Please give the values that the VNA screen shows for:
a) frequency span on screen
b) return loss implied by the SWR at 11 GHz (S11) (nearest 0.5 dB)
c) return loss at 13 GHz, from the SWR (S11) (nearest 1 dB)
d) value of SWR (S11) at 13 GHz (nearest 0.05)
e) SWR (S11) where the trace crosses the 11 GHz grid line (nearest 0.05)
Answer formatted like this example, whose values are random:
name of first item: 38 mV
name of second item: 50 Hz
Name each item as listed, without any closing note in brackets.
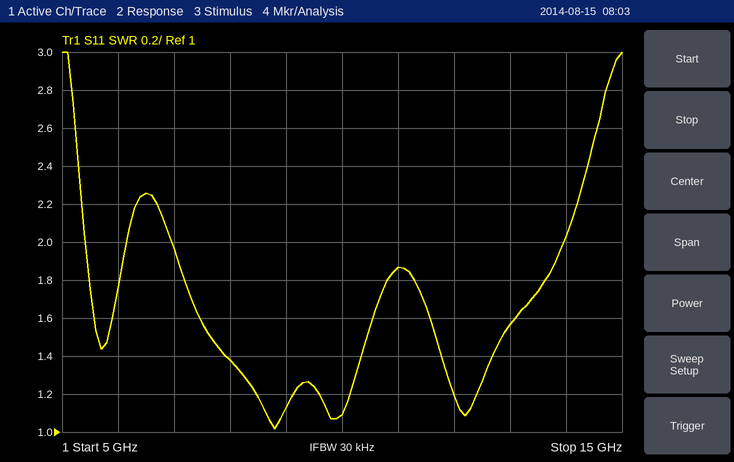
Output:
frequency span on screen: 10 GHz
return loss implied by the SWR at 11 GHz (S11): 10.5 dB
return loss at 13 GHz, from the SWR (S11): 13 dB
value of SWR (S11) at 13 GHz: 1.55
SWR (S11) where the trace crosses the 11 GHz grid line: 1.85
